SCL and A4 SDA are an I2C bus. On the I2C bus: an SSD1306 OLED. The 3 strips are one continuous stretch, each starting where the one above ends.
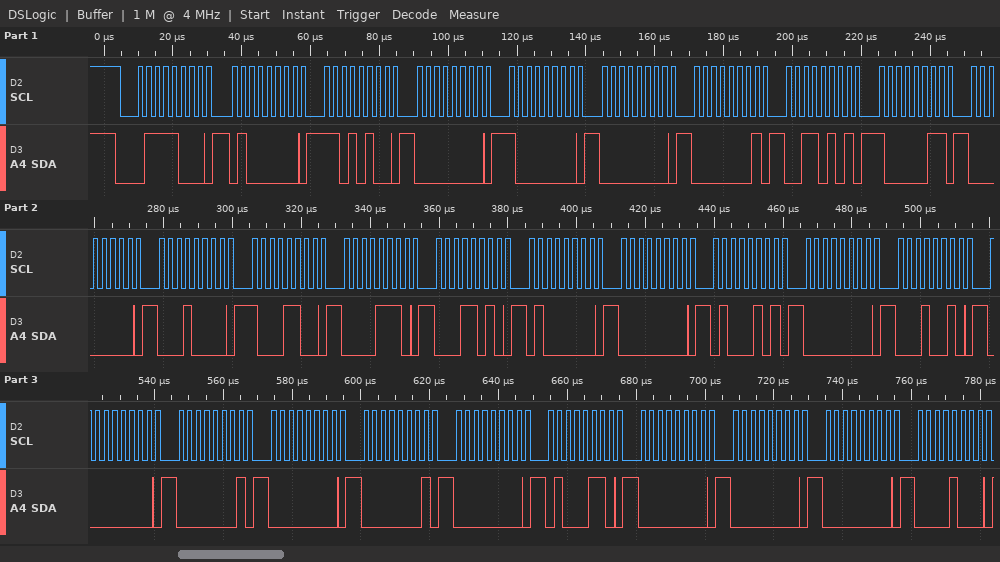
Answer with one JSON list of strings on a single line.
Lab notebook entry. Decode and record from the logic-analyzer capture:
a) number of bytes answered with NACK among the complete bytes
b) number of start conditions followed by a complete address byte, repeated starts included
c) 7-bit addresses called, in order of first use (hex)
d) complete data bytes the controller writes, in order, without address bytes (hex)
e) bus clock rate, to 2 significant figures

["0", "1", "0x3C", "40 D4 00 80 00 01 35 83 00 10 8C 0E 1A 40 00 45 00 12 00 01 00 01 00 46 00 00 00 08", "400 kHz"]
